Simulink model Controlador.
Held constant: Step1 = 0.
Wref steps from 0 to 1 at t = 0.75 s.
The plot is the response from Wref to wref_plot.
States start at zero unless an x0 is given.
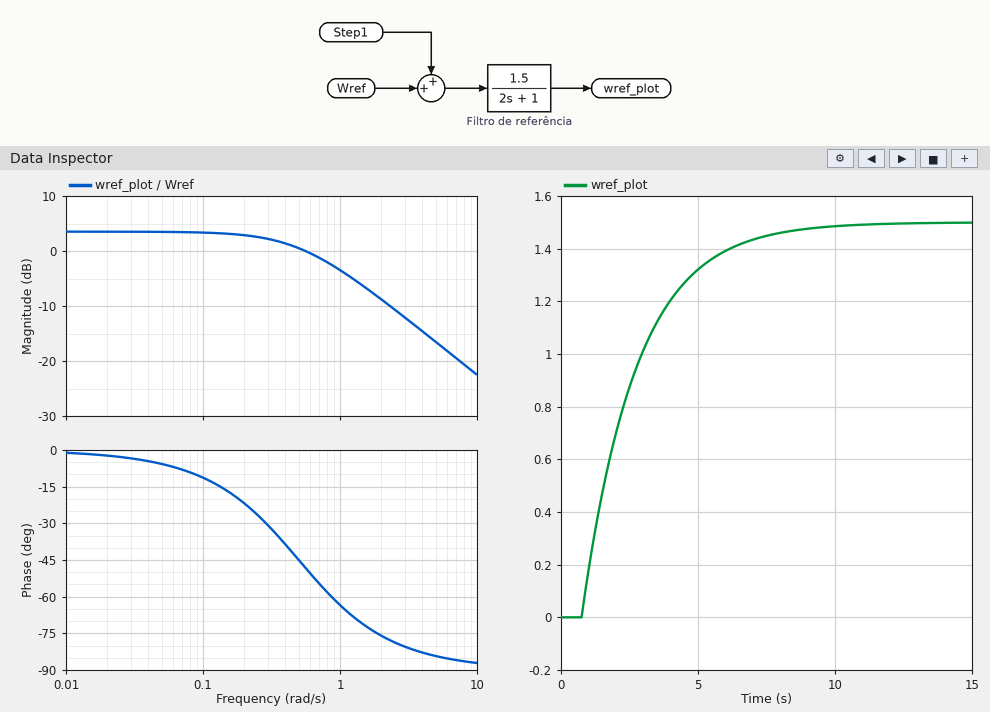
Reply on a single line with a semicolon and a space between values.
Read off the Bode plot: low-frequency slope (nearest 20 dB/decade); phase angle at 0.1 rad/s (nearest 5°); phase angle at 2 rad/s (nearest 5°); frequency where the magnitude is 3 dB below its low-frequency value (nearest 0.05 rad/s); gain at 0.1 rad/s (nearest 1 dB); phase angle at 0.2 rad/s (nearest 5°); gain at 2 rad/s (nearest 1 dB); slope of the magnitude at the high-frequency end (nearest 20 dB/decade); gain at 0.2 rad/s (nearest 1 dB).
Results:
0 dB/decade; -10°; -75°; 0.50 rad/s; 3 dB; -20°; -9 dB; -20 dB/decade; 3 dB
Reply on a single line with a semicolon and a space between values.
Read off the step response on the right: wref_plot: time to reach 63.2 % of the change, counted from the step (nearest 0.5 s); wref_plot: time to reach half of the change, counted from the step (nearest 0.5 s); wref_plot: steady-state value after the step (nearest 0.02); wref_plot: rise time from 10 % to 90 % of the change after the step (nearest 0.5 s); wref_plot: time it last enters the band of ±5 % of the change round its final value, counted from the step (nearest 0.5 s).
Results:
2.0 s; 1.5 s; 1.50; 4.5 s; 6.0 s
